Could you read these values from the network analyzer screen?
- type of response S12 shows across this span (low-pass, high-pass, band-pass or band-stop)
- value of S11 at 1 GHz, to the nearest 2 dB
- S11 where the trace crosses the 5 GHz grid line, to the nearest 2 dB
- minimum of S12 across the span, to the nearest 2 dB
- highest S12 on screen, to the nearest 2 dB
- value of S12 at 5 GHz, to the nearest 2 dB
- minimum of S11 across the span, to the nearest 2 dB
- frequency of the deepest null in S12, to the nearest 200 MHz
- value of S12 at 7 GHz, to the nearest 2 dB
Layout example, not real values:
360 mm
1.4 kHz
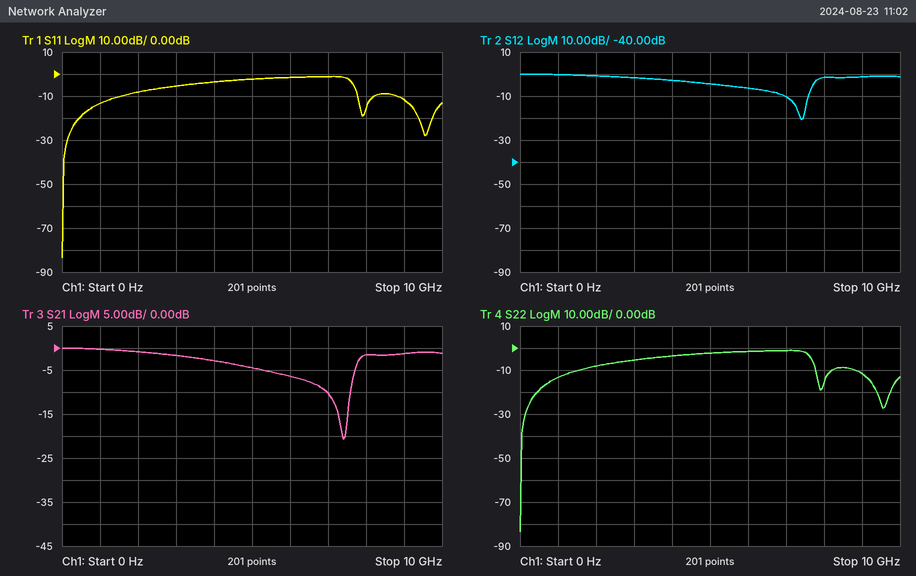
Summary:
band-stop
-14 dB
-2 dB
-20 dB
0 dB
-4 dB
-84 dB
7.4 GHz
-10 dB
